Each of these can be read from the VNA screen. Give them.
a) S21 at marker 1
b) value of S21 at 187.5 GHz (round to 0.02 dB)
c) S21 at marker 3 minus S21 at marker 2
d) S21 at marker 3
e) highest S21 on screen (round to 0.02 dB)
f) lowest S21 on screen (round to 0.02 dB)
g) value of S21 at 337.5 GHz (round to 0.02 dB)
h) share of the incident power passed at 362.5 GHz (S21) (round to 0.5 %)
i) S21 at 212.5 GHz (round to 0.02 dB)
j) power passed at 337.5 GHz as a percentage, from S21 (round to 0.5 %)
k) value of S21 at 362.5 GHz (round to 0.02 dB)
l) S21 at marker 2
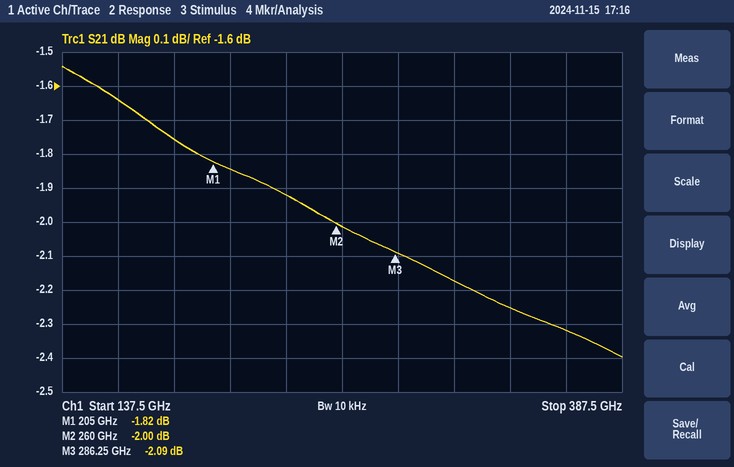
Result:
-1.82 dB
-1.76 dB
-0.09 dB
-2.09 dB
-1.54 dB
-2.40 dB
-2.26 dB
58.5 %
-1.84 dB
59.5 %
-2.32 dB
-2.00 dB
